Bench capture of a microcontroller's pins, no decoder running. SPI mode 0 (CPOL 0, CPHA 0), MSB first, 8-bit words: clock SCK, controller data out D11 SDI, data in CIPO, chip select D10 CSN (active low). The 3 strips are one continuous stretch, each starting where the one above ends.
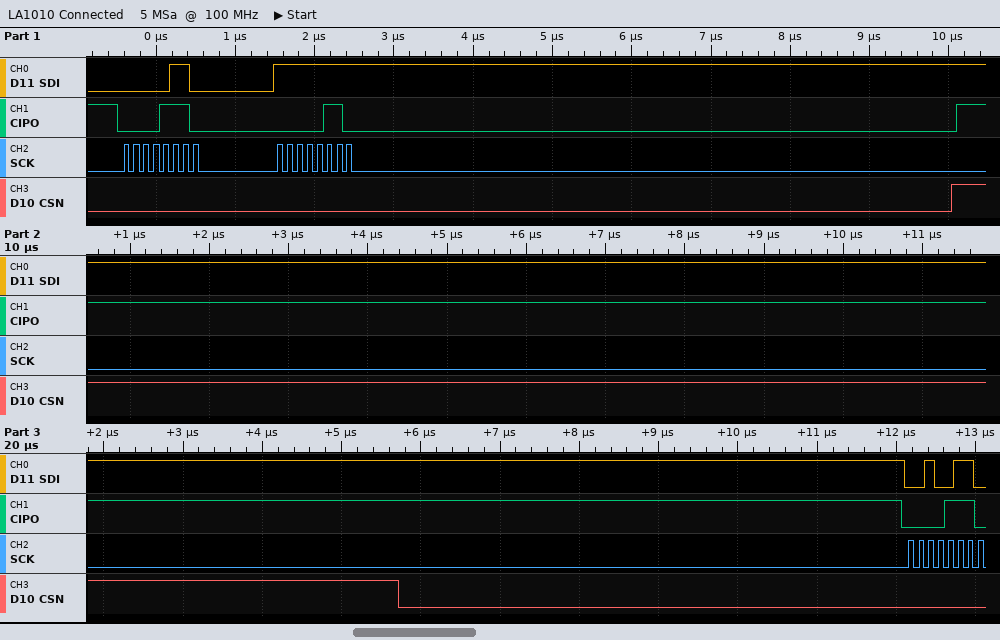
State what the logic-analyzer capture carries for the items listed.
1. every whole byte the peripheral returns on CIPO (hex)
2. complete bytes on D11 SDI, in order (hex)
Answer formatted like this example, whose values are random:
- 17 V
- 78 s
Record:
- 0x0E 0x06 0x0E
- 0x06 0xFF 0x26
